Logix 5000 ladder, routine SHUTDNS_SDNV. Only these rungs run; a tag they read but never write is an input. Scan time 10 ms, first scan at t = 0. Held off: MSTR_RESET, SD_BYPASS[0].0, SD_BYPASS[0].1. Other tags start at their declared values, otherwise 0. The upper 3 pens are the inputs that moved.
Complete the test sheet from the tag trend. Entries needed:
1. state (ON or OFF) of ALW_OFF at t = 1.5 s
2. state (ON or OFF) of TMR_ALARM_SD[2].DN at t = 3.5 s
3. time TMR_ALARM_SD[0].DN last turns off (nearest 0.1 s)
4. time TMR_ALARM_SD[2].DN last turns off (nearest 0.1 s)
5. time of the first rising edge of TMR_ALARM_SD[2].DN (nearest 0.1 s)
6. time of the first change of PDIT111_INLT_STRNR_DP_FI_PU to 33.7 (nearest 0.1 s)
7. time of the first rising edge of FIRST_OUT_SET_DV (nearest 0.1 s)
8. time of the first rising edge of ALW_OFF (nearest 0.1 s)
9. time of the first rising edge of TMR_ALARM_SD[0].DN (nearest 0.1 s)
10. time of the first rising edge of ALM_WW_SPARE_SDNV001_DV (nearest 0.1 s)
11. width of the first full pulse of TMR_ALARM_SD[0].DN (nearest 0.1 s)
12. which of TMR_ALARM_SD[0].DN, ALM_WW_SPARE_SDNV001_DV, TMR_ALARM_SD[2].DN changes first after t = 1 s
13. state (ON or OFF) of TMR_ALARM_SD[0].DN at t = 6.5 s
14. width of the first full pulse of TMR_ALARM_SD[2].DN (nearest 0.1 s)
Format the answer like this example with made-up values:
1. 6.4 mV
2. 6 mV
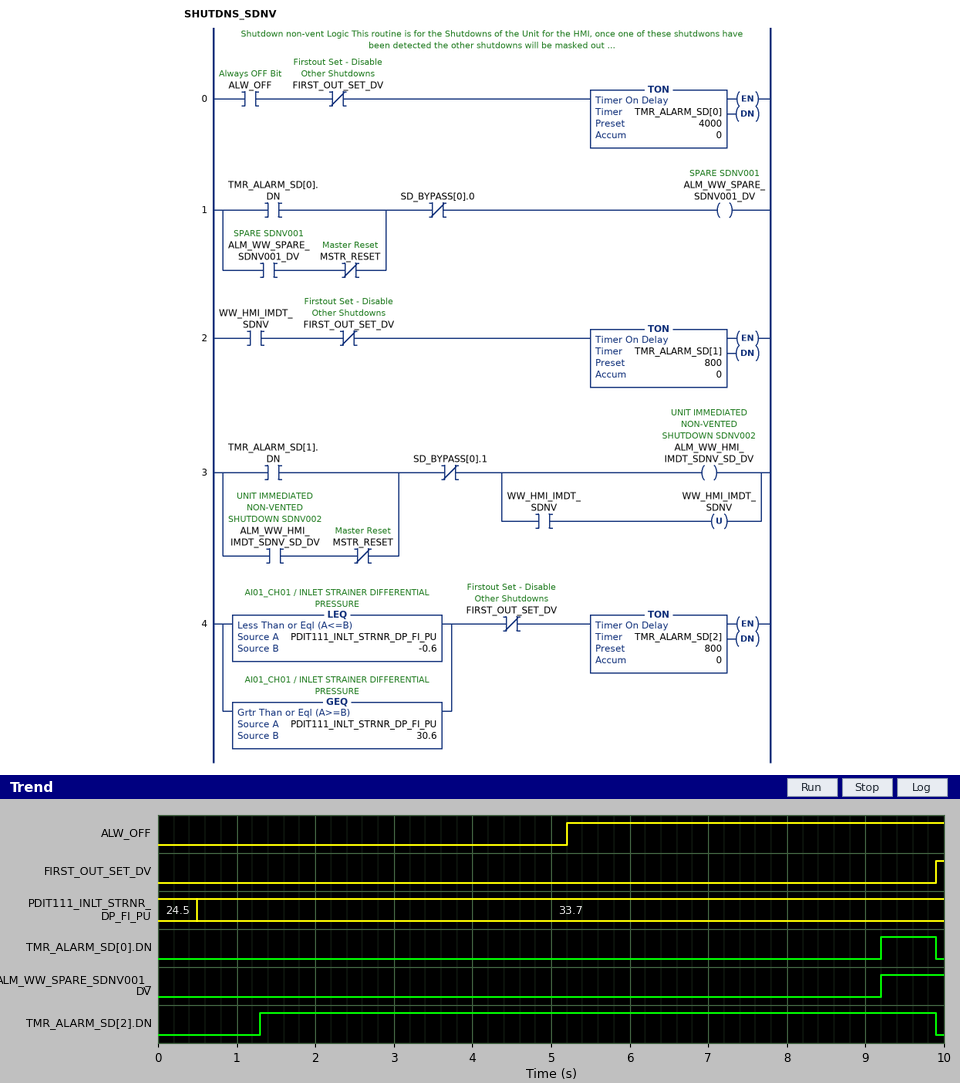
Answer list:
1. OFF
2. ON
3. 9.9 s
4. 9.9 s
5. 1.3 s
6. 0.5 s
7. 9.9 s
8. 5.2 s
9. 9.2 s
10. 9.2 s
11. 0.7 s
12. TMR_ALARM_SD[2].DN
13. OFF
14. 8.6 s
